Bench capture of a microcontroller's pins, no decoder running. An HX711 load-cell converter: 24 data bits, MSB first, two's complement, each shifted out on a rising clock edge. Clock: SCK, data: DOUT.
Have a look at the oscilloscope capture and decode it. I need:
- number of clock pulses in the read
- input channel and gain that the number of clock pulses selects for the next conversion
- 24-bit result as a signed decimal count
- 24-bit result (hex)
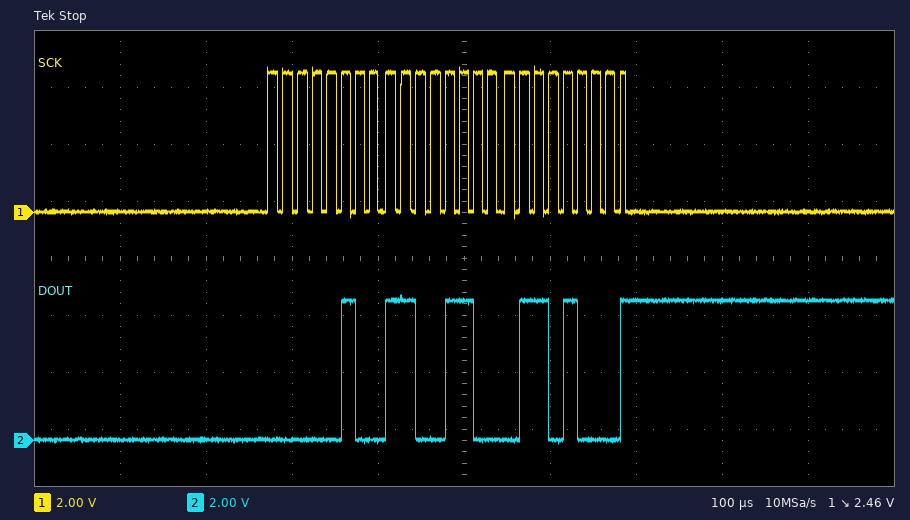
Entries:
25
channel A, gain 128
314472
0x04CC68
